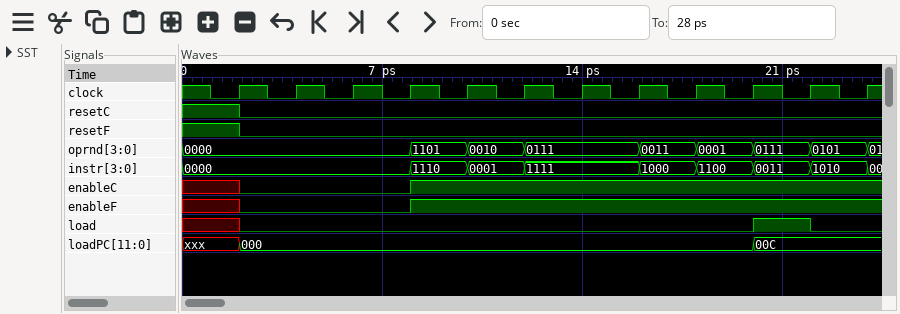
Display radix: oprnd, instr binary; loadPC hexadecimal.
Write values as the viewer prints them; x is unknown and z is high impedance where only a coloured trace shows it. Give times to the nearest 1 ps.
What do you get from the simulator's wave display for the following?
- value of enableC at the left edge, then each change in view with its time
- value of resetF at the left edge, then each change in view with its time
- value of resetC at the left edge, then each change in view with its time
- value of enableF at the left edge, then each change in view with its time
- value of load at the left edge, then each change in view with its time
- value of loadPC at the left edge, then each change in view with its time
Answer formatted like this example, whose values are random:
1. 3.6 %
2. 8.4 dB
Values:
1. x, 0 at 2 ps, 1 at 8 ps
2. 1, 0 at 2 ps
3. 1, 0 at 2 ps
4. x, 0 at 2 ps, 1 at 8 ps
5. x, 0 at 2 ps, 1 at 20 ps, 0 at 22 ps
6. xxx, 000 at 2 ps, 00C at 20 ps
